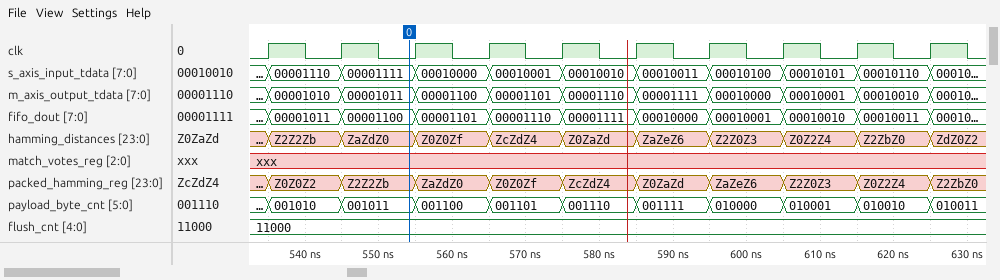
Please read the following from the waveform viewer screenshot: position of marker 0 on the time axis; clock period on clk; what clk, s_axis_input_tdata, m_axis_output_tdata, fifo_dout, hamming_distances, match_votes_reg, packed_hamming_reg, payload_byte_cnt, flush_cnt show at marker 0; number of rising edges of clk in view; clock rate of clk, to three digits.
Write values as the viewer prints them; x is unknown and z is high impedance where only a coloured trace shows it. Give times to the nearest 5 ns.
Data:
555 ns
10 ns
clk=0, s_axis_input_tdata=00001111, m_axis_output_tdata=00001011, fifo_dout=00001100, hamming_distances=ZaZdZ0, match_votes_reg=xxx, packed_hamming_reg=Z2Z2Zb, payload_byte_cnt=001011, flush_cnt=11000
10
100 MHz
